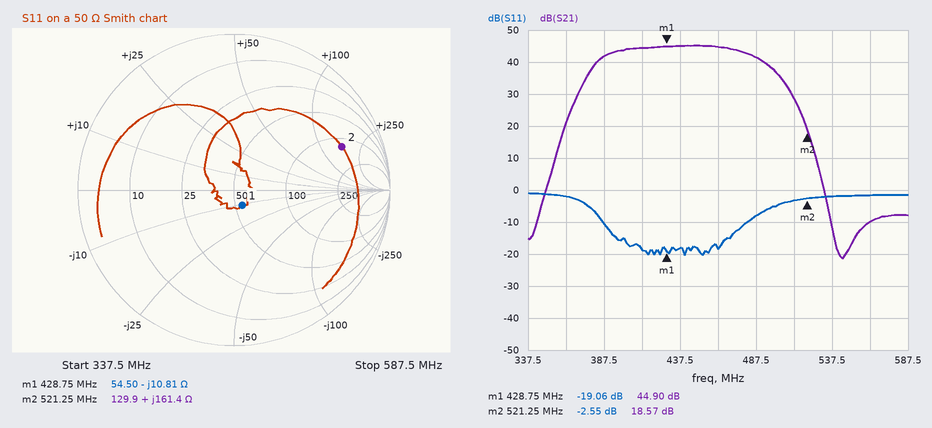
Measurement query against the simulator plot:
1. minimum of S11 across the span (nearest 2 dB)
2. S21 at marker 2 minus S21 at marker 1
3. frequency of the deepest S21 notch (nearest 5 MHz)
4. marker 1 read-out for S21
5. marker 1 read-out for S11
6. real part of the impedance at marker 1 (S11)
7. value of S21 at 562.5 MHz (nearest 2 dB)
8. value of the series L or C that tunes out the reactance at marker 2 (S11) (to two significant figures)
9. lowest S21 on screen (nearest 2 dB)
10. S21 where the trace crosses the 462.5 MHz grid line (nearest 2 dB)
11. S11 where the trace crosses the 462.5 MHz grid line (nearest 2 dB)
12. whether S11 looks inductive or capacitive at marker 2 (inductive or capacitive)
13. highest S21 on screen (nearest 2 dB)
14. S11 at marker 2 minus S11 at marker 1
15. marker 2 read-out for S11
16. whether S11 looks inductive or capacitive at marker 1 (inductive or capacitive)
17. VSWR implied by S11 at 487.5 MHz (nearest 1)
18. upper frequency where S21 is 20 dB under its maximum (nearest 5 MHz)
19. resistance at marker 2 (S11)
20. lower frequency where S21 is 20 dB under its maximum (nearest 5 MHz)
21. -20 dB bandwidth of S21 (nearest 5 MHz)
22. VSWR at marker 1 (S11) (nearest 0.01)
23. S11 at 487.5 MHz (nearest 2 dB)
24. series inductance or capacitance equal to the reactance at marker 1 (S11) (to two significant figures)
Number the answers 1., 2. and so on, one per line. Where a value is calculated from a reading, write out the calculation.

1. -20 dB
2. 18.57 − (44.9) = -26.33 dB
3. 545 MHz
4. 44.90 dB
5. -19.06 dB
6. 54.50 Ω
7. -10 dB
8. C = 1/(2π × 521.25 MHz × 161.4 Ω) ≈ 1.9 pF
9. -22 dB
10. 44 dB
11. -18 dB
12. inductive
13. 46 dB
14. -2.55 − (-19.06) = 16.51 dB
15. -2.55 dB
16. capacitive
17. |Γ| = 10^(-8/20) = 0.3981; VSWR = (1 + 0.3981)/(1 − 0.3981) ≈ 2
18. 515 MHz
19. 129.9 Ω
20. 365 MHz
21. 515 MHz − 365 MHz = 150 MHz
22. 1.25
23. -8 dB
24. C = 1/(2π × 428.75 MHz × 10.81 Ω) ≈ 34 pF
